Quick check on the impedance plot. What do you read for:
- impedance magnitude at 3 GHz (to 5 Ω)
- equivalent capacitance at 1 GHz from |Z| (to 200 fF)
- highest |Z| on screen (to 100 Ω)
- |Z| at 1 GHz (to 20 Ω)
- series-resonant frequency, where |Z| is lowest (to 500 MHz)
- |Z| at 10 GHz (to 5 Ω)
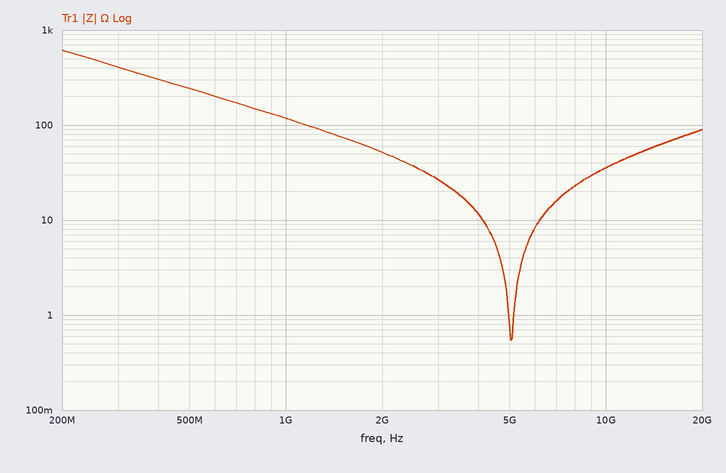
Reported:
25 Ω
1.4 pF
600 Ω
120 Ω
5.0 GHz
35 Ω
